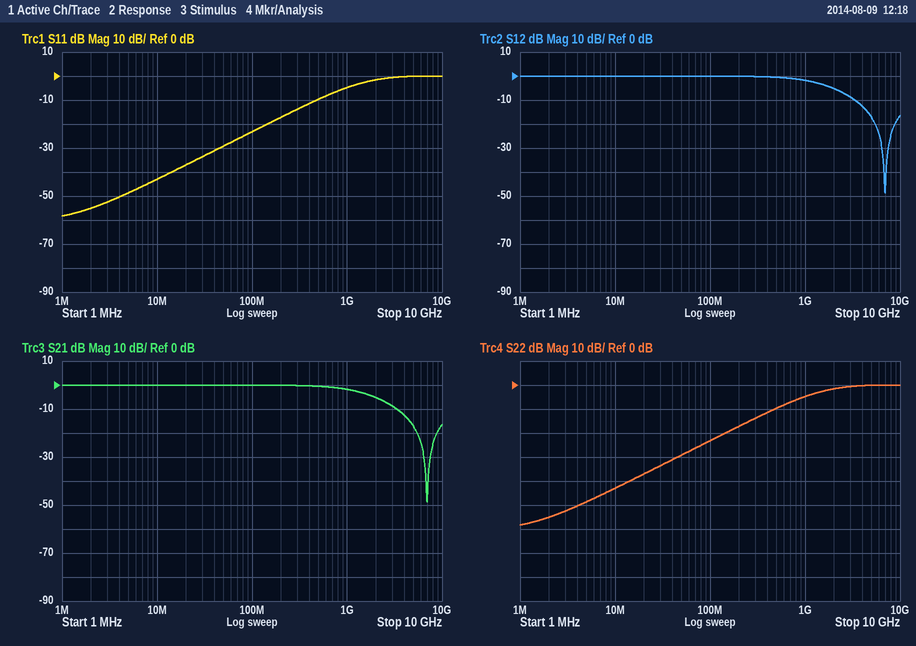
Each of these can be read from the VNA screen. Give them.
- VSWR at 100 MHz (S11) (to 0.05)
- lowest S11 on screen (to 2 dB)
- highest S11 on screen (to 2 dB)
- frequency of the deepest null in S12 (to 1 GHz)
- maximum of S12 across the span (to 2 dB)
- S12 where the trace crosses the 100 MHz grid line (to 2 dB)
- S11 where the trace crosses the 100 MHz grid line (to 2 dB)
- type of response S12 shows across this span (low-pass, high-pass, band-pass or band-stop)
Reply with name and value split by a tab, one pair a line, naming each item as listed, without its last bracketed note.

VSWR at 100 MHz (S11)	1.15
lowest S11 on screen	-58 dB
highest S11 on screen	0 dB
frequency of the deepest null in S12	7 GHz
maximum of S12 across the span	0 dB
S12 where the trace crosses the 100 MHz grid line	0 dB
S11 where the trace crosses the 100 MHz grid line	-24 dB
type of response S12 shows across this span	low-pass
